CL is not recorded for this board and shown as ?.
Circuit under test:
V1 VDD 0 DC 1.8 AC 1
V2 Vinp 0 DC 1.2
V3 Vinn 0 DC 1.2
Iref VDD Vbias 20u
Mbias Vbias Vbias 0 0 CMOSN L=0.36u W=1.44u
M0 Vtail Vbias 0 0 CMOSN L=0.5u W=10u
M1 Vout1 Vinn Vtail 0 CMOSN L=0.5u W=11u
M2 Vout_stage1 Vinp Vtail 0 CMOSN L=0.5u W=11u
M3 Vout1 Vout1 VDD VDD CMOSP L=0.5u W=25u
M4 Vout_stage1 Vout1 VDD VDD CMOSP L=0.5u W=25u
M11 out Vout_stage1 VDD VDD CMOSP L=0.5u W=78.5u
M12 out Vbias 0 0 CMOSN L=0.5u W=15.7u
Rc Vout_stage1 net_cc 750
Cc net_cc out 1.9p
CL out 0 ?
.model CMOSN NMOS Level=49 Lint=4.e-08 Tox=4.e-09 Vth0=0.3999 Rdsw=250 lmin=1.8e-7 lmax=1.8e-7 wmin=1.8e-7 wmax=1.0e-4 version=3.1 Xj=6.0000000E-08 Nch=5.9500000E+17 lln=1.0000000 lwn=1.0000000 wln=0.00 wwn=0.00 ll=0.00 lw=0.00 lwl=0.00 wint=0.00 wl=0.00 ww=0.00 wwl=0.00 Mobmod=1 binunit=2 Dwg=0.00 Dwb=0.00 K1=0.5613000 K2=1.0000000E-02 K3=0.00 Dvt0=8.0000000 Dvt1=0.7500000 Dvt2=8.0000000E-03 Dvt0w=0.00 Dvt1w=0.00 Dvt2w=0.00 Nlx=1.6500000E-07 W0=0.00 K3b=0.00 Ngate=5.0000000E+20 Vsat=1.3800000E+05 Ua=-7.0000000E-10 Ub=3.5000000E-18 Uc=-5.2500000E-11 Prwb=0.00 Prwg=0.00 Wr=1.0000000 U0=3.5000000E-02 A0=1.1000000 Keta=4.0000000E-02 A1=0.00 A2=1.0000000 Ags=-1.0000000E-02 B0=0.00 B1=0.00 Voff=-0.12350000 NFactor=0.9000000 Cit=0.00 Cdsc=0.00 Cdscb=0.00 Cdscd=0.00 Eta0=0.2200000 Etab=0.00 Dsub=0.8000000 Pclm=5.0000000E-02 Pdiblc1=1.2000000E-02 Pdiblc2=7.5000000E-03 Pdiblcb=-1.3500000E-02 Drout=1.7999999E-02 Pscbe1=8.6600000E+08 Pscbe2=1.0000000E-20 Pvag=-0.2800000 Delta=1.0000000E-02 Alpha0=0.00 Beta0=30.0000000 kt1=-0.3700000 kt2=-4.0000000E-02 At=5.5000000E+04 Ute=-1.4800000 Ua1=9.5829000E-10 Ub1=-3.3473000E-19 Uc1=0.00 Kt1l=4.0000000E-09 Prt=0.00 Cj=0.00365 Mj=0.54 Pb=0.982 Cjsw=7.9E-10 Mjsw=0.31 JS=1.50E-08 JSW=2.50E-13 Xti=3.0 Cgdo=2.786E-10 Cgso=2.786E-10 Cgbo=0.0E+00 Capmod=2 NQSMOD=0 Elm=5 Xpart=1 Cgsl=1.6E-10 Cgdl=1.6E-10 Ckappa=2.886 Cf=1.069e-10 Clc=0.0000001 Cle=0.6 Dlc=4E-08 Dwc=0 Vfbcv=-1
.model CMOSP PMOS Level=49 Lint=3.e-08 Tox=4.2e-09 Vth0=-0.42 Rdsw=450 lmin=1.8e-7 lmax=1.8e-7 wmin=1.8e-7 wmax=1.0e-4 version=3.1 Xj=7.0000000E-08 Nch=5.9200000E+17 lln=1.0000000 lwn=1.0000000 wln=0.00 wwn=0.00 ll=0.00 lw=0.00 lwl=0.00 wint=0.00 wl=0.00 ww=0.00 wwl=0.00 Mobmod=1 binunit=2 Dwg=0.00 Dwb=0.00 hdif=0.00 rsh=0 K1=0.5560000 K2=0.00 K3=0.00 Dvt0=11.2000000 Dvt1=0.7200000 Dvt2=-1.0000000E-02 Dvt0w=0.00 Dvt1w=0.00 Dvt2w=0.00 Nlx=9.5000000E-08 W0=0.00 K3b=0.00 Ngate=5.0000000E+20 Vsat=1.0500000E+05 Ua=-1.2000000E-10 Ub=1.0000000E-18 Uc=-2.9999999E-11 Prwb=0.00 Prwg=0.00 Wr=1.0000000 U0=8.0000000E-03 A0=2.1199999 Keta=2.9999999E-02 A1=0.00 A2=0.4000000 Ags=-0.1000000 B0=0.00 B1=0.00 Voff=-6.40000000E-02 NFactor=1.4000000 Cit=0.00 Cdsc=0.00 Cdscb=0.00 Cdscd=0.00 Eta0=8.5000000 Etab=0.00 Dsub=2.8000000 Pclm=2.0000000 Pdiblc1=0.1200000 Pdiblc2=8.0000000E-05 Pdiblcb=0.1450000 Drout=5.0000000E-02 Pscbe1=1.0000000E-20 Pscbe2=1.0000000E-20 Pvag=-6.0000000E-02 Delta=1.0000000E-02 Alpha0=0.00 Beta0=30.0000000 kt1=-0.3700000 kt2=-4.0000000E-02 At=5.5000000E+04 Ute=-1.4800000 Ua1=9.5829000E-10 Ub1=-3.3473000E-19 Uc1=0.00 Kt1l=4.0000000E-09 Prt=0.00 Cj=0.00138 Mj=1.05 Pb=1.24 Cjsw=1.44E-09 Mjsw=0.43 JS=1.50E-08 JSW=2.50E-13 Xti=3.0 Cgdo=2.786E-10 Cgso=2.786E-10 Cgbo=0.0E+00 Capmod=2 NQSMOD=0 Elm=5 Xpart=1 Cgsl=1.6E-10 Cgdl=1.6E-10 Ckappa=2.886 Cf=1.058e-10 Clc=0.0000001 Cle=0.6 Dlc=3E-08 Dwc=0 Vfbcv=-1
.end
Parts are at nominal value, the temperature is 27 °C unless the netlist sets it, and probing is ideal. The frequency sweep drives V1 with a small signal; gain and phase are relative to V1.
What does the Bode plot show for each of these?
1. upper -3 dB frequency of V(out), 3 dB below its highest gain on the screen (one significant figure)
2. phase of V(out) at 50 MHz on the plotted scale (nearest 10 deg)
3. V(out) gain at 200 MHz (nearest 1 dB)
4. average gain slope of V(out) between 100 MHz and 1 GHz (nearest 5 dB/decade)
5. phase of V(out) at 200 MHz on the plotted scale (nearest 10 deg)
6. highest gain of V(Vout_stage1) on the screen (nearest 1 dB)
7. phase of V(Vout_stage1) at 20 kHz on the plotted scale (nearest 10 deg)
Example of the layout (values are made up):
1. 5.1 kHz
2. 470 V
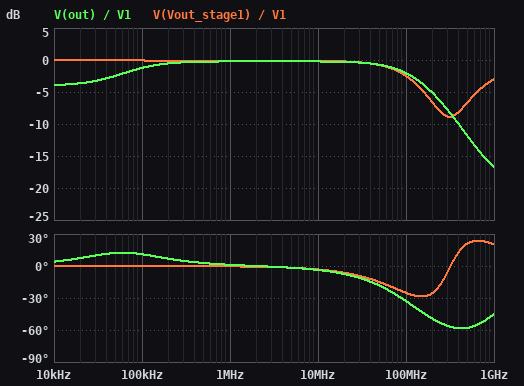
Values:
1. 100 MHz
2. -20 deg
3. -5 dB
4. -15 dB/decade
5. -50 deg
6. 0 dB
7. 0 deg
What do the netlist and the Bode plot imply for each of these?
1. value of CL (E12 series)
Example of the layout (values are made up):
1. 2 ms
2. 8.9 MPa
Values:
1. 1.8 pF
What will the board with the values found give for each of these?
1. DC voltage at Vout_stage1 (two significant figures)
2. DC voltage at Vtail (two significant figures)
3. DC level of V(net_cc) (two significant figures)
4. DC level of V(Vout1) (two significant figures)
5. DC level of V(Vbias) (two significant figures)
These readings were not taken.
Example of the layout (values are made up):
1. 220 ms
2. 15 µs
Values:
1. 1.1 V
2. 460 mV
3. 1.1 V
4. 1.1 V
5. 690 mV
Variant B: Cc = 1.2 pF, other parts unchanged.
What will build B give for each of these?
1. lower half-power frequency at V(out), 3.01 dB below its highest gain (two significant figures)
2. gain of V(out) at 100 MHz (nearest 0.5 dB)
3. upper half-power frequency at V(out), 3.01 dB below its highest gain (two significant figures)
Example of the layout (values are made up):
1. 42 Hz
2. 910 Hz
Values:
1. 46 kHz
2. -2.5 dB
3. 130 MHz
